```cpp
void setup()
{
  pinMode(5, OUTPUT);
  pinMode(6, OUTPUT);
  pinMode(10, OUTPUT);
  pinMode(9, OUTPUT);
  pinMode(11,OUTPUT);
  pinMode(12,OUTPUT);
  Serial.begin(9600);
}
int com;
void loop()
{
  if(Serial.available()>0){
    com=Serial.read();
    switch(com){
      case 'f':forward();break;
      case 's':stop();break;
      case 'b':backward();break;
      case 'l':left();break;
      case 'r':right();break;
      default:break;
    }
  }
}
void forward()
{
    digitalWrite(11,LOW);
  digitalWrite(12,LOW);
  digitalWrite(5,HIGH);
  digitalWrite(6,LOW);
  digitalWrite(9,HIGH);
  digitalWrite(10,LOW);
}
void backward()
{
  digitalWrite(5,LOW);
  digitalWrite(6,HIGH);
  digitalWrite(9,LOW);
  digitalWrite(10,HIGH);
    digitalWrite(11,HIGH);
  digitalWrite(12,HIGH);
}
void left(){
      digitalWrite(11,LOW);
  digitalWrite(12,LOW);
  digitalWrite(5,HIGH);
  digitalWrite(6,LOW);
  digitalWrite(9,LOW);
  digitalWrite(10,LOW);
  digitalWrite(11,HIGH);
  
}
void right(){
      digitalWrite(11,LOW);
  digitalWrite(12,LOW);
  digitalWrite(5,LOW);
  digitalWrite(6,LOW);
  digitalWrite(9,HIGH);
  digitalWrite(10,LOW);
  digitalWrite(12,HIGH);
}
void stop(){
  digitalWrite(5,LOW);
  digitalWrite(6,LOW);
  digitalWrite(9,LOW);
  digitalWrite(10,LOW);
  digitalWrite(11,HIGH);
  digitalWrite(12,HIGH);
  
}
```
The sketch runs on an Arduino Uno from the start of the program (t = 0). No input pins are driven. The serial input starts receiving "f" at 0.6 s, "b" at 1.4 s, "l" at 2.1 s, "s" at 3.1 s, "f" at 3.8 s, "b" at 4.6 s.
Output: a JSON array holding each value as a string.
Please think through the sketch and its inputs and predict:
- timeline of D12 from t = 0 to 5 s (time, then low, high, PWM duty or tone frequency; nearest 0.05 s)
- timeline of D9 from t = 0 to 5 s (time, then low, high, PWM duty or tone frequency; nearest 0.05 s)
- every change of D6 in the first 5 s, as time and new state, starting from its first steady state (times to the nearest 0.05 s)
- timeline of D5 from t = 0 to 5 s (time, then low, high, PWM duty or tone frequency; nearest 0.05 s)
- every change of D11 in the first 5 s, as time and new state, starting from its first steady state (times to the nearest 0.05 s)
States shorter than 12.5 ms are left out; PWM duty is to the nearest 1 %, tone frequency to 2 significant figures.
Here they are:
["0 s low; 1.4 s high; 2.1 s low; 3.1 s high; 3.8 s low; 4.6 s high", "0 s low; 0.6 s high; 1.4 s low; 3.8 s high; 4.6 s low", "0 s low; 1.4 s high; 2.1 s low; 4.6 s high", "0 s low; 0.6 s high; 1.4 s low; 2.1 s high; 3.1 s low; 3.8 s high; 4.6 s low", "0 s low; 1.4 s high; 3.8 s low; 4.6 s high"]
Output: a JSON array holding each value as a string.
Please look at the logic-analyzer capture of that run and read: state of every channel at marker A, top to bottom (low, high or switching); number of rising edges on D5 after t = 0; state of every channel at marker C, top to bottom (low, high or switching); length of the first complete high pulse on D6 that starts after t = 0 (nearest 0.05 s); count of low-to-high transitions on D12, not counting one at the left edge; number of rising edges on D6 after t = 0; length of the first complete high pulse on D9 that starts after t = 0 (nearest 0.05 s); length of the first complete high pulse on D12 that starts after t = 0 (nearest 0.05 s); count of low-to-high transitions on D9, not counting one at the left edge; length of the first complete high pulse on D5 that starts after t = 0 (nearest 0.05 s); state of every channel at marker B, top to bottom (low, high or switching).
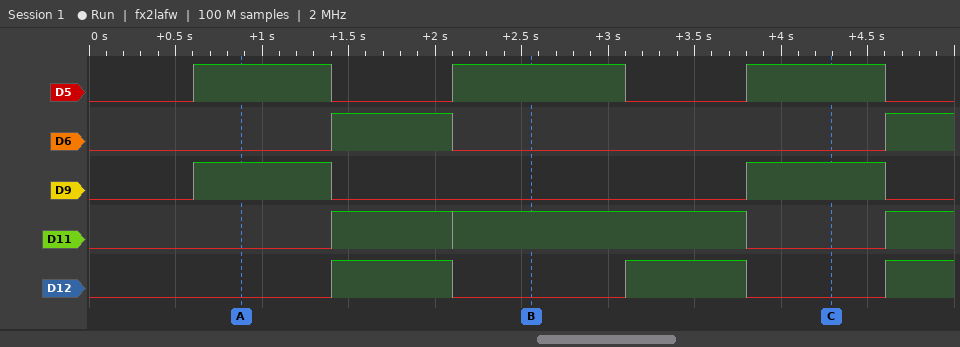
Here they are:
["D5 high, D6 low, D9 high, D11 low, D12 low", "3", "D5 high, D6 low, D9 high, D11 low, D12 low", "0.70 s", "3", "2", "0.80 s", "0.70 s", "2", "0.80 s", "D5 high, D6 low, D9 low, D11 high, D12 low"]
